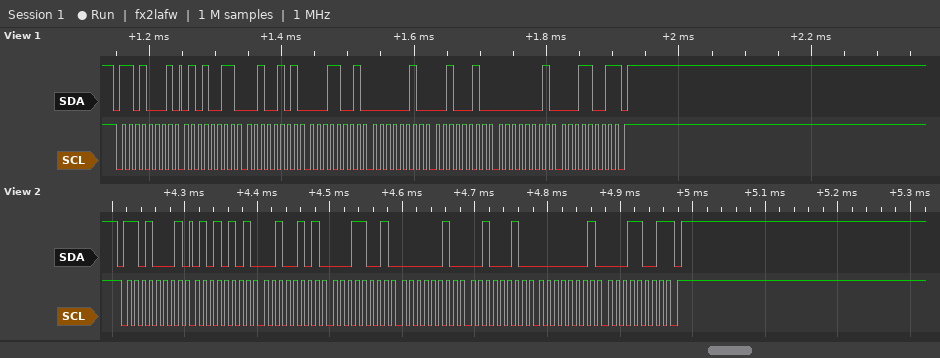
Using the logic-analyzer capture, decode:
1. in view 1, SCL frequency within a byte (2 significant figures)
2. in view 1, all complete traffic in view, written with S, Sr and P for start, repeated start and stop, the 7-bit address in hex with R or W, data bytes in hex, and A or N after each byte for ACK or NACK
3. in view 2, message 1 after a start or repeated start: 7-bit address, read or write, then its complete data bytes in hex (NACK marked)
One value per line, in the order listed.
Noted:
100 kHz
S 68R A 53 A 25 A 19 A 02 A 22 A 01 A 19 N P
0x68 read: 55 25 19 02 22 01 19 NACK
